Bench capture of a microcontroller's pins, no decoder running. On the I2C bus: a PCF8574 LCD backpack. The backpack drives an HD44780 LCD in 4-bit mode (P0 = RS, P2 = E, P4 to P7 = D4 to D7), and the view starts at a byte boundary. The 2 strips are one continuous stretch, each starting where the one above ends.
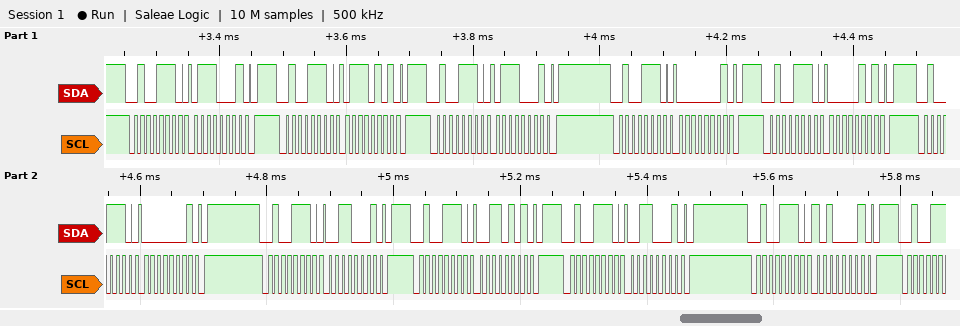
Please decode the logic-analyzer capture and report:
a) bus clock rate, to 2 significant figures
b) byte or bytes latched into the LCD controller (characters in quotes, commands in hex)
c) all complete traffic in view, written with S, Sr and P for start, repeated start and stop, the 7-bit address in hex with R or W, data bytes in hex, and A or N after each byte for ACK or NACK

100 kHz
'p'
S 27W A 71 A P S 27W A 75 A P S 27W A 71 A P S 27W A 01 A P S 27W A 05 A P S 27W A 01 A P S 27W A 31 A P S 27W A 35 A P S 27W A 31 A P S 27W A A1 A P
